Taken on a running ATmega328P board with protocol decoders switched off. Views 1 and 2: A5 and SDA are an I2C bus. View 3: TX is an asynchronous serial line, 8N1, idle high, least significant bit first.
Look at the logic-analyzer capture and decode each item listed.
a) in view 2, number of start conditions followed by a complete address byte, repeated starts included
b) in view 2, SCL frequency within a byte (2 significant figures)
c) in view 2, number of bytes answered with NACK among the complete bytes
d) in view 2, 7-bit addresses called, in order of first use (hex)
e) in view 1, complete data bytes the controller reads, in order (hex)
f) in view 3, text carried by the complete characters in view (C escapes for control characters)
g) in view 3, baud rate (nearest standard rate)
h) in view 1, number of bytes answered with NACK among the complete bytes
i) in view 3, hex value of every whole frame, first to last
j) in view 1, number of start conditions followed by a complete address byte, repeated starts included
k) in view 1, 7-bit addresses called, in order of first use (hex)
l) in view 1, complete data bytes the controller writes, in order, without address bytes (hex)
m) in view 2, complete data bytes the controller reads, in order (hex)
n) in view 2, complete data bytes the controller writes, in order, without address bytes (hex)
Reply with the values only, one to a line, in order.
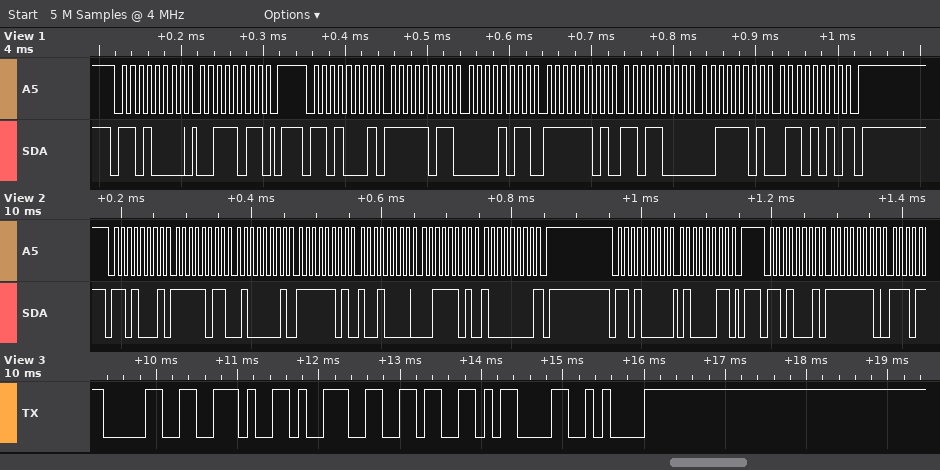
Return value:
3
100 kHz
1
0x68
FB 0B FD D8 3D 6A
"0.96\r\n"
9600 baud
1
30 2E 39 36 0D 0A
2
0x68
3B
FB 41 FD 90 3D 80 FE
43
